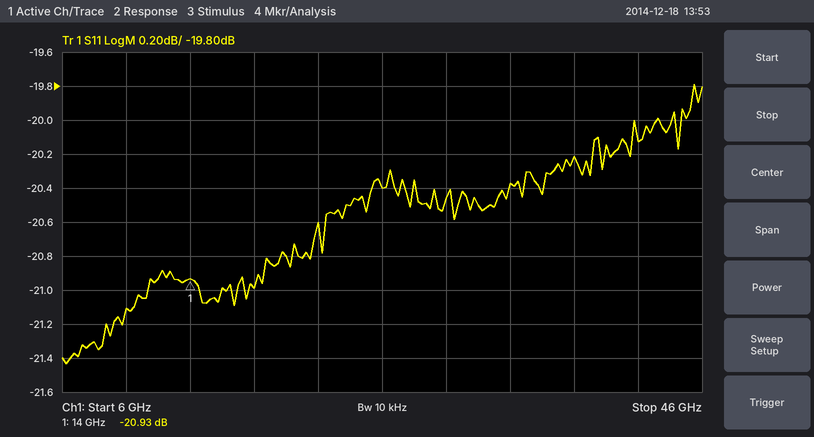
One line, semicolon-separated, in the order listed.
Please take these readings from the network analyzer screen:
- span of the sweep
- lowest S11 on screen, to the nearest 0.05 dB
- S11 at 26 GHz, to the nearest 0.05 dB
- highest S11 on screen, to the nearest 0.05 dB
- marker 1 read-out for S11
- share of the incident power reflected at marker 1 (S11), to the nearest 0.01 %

40 GHz; -21.45 dB; -20.40 dB; -19.80 dB; -20.93 dB; 0.81 %
